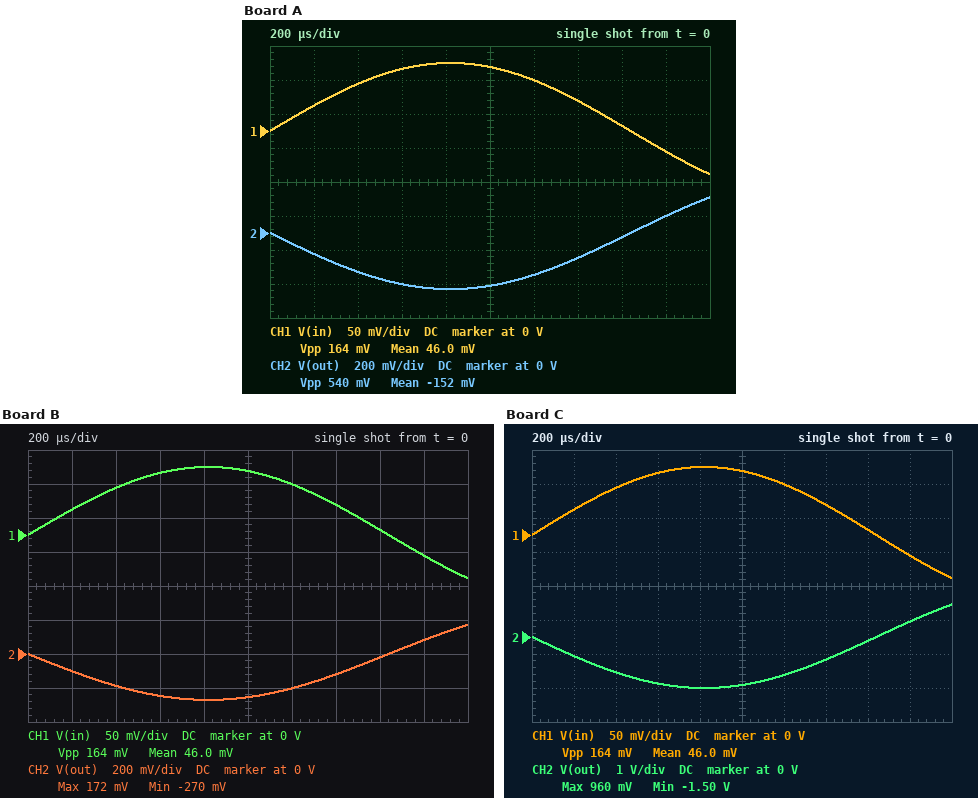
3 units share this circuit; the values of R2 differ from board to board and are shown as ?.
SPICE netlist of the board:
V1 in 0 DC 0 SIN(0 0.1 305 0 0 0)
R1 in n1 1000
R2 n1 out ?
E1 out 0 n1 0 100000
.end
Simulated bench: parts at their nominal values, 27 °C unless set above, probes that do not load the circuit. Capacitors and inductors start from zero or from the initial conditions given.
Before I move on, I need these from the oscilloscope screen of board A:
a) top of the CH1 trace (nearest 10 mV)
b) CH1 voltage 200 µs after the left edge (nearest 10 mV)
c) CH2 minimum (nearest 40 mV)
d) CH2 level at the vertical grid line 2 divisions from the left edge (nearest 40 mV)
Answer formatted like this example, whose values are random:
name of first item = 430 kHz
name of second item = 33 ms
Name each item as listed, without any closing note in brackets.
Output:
top of the CH1 trace = 100 mV
CH1 voltage 200 µs after the left edge = 40 mV
CH2 minimum = -320 mV
CH2 level at the vertical grid line 2 divisions from the left edge = -240 mV
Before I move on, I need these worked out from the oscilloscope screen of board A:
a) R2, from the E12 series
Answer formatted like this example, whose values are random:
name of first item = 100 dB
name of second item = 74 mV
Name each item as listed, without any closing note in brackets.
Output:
R2, from the E12 series = 3.3 kΩ
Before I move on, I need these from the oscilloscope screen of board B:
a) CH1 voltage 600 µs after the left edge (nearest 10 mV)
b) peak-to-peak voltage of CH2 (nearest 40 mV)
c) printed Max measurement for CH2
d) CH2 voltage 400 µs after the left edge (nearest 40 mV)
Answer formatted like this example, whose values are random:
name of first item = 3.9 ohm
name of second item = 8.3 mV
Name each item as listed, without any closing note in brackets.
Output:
CH1 voltage 600 µs after the left edge = 90 mV
peak-to-peak voltage of CH2 = 440 mV
printed Max measurement for CH2 = 172 mV
CH2 voltage 400 µs after the left edge = -200 mV
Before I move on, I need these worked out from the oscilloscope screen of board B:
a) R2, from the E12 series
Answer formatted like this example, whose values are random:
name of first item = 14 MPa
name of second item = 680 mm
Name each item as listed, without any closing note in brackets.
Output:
R2, from the E12 series = 2.7 kΩ
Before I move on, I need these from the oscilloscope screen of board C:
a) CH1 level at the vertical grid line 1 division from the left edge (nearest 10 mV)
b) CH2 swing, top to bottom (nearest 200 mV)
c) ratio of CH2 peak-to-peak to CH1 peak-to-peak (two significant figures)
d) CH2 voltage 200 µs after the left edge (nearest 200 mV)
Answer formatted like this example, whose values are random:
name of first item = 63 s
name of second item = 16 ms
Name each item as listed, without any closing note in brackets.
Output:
CH1 level at the vertical grid line 1 division from the left edge = 40 mV
CH2 swing, top to bottom = 2.4 V
ratio of CH2 peak-to-peak to CH1 peak-to-peak = 15
CH2 voltage 200 µs after the left edge = -600 mV
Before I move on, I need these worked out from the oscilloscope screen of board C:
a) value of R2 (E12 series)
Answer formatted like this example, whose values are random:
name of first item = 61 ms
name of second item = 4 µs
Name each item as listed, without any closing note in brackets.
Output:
value of R2 = 15 kΩ
